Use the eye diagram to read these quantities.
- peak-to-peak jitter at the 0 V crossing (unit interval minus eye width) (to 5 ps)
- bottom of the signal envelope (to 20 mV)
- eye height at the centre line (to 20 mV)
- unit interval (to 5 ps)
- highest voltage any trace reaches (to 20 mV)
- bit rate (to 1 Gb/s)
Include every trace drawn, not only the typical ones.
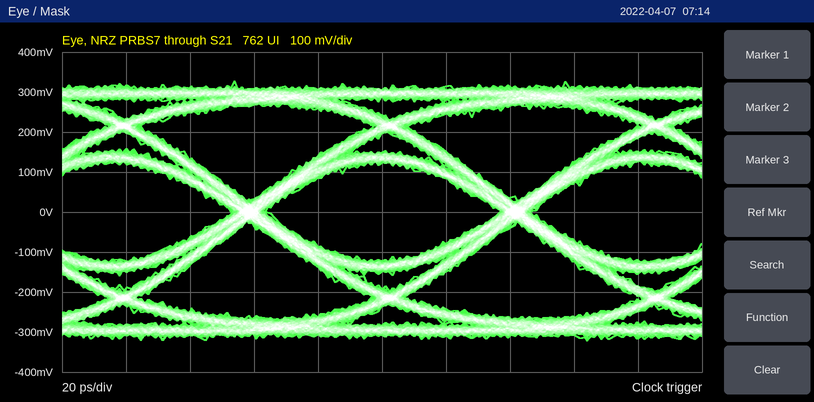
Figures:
10 ps
-320 mV
240 mV
85 ps
320 mV
12 Gb/s
